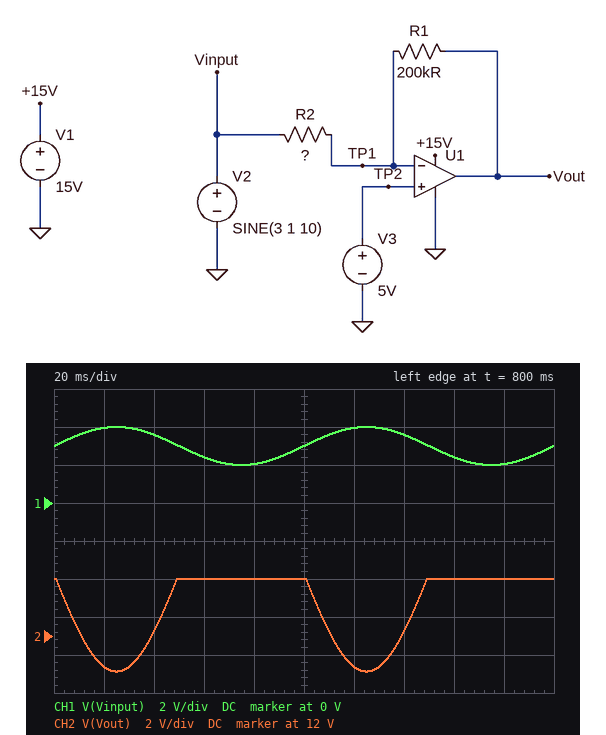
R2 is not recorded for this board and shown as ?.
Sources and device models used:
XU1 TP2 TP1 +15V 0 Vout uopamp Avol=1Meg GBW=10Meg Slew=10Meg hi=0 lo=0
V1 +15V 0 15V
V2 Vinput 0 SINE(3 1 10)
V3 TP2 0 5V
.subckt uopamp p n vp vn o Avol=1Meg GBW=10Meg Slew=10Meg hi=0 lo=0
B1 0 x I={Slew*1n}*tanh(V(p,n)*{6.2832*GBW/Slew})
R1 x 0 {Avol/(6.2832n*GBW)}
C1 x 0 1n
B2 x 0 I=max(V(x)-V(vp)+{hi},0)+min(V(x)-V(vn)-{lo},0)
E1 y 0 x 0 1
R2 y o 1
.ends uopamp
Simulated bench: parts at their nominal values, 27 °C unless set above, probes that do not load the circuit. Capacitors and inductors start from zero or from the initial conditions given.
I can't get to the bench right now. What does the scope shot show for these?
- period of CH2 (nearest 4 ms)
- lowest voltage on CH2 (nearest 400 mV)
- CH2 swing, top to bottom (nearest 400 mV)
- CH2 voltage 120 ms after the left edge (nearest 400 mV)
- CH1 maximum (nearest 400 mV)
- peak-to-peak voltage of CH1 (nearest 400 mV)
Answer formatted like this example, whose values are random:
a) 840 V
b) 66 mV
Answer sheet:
a) 100 ms
b) 10.0 V
c) 4.8 V
d) 10.4 V
e) 4.0 V
f) 2.0 V
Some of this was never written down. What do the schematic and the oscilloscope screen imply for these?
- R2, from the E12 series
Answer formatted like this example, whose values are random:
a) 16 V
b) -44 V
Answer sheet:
a) 39 kΩ
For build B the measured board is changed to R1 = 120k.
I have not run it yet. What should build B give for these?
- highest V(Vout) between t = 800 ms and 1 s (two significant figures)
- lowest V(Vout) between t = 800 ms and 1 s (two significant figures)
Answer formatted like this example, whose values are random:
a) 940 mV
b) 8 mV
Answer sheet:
a) 14 V
b) 8.1 V
